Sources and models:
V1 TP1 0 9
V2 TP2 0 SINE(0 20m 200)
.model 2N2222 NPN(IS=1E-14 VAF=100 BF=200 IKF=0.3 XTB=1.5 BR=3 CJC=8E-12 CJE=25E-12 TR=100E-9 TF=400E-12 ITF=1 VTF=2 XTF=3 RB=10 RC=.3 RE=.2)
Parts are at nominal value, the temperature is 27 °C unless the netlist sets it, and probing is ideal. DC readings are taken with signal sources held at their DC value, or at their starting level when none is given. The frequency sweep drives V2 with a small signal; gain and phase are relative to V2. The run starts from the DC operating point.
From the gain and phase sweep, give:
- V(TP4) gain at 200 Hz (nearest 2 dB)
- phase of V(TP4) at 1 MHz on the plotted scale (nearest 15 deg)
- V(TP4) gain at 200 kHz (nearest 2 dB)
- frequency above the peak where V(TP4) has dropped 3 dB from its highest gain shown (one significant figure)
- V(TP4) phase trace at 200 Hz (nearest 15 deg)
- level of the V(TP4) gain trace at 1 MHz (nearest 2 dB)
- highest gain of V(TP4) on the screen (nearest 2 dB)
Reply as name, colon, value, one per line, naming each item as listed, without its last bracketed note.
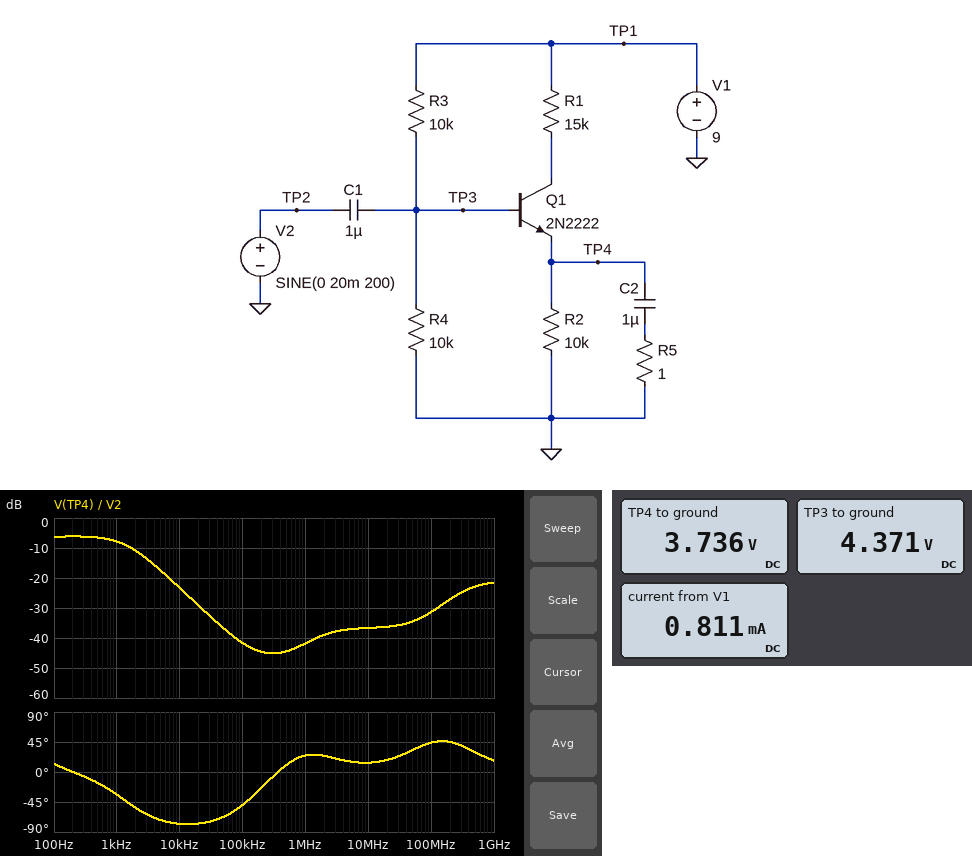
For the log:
V(TP4) gain at 200 Hz: -6 dB
phase of V(TP4) at 1 MHz on the plotted scale: 30 deg
V(TP4) gain at 200 kHz: -44 dB
frequency above the peak where V(TP4) has dropped 3 dB from its highest gain shown: 1 kHz
V(TP4) phase trace at 200 Hz: 0 deg
level of the V(TP4) gain trace at 1 MHz: -42 dB
highest gain of V(TP4) on the screen: -6 dB
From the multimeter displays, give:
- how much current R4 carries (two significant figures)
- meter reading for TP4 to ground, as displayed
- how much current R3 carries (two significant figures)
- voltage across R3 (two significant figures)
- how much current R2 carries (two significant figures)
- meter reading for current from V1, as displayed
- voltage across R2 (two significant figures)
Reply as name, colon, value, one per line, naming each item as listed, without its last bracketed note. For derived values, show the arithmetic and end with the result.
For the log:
how much current R4 carries: (4.371 V) / 10 kΩ = 440 µA
meter reading for TP4 to ground, as displayed: 3.736 V
how much current R3 carries: (9 V - 4.371 V) / 10 kΩ = 460 µA
voltage across R3: 9 V - 4.371 V = 4.6 V
how much current R2 carries: (3.736 V) / 10 kΩ = 370 µA
meter reading for current from V1, as displayed: 0.811 mA
voltage across R2: 3.736 V = 3.7 V
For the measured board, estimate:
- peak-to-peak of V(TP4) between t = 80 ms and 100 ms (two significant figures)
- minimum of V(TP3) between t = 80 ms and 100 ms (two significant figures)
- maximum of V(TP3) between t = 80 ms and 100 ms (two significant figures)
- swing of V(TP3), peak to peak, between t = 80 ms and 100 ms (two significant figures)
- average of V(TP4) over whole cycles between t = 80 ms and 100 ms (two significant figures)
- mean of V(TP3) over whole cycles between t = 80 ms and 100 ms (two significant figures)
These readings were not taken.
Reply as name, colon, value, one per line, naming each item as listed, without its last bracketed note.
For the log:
peak-to-peak of V(TP4) between t = 80 ms and 100 ms: 20 mV
minimum of V(TP3) between t = 80 ms and 100 ms: 4.4 V
maximum of V(TP3) between t = 80 ms and 100 ms: 4.4 V
swing of V(TP3), peak to peak, between t = 80 ms and 100 ms: 21 mV
average of V(TP4) over whole cycles between t = 80 ms and 100 ms: 3.7 V
mean of V(TP3) over whole cycles between t = 80 ms and 100 ms: 4.4 V
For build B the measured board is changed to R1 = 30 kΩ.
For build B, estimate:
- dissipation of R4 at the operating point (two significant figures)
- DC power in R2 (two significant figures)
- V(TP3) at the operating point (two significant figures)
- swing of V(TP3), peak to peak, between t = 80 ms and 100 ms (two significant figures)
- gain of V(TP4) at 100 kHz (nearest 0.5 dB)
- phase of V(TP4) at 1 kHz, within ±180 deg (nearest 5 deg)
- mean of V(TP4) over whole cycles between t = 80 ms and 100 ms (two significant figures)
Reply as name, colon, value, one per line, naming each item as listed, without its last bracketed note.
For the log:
dissipation of R4 at the operating point: 1.5 mW
DC power in R2: 1.0 mW
V(TP3) at the operating point: 3.9 V
swing of V(TP3), peak to peak, between t = 80 ms and 100 ms: 20 mV
gain of V(TP4) at 100 kHz: -38.5 dB
phase of V(TP4) at 1 kHz, within ±180 deg: -25 deg
mean of V(TP4) over whole cycles between t = 80 ms and 100 ms: 3.2 V
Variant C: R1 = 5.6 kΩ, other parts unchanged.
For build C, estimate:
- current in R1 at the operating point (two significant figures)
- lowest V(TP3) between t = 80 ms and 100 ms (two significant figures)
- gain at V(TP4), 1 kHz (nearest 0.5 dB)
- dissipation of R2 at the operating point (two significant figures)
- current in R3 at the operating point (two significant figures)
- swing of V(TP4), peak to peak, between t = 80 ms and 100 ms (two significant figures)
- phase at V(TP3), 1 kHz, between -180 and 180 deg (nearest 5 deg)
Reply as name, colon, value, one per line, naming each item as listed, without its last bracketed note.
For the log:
current in R1 at the operating point: 380 µA
lowest V(TP3) between t = 80 ms and 100 ms: 4.5 V
gain at V(TP4), 1 kHz: -1.0 dB
dissipation of R2 at the operating point: 1.5 mW
current in R3 at the operating point: 450 µA
swing of V(TP4), peak to peak, between t = 80 ms and 100 ms: 39 mV
phase at V(TP3), 1 kHz, between -180 and 180 deg: 0 deg
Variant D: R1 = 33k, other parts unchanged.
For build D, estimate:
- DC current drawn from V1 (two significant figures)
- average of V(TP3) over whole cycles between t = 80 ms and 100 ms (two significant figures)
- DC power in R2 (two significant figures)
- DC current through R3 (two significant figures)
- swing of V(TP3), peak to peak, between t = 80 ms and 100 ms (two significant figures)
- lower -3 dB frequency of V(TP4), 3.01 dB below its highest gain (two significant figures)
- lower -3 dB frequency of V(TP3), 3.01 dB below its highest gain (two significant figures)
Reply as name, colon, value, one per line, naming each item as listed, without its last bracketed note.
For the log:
DC current drawn from V1: 700 µA
average of V(TP3) over whole cycles between t = 80 ms and 100 ms: 3.8 V
DC power in R2: 1.0 mW
DC current through R3: 520 µA
swing of V(TP3), peak to peak, between t = 80 ms and 100 ms: 20 mV
lower -3 dB frequency of V(TP4), 3.01 dB below its highest gain: 26 Hz
lower -3 dB frequency of V(TP3), 3.01 dB below its highest gain: 1.5 kHz
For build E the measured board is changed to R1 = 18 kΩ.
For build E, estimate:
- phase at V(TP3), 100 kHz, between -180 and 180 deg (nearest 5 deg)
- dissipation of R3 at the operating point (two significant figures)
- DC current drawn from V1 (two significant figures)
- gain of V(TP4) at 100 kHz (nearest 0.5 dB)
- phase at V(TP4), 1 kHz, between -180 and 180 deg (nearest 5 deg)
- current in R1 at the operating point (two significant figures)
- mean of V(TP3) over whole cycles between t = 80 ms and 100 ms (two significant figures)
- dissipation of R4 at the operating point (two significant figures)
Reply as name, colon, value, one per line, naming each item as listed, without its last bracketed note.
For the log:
phase at V(TP3), 100 kHz, between -180 and 180 deg: 0 deg
dissipation of R3 at the operating point: 2.3 mW
DC current drawn from V1: 780 µA
gain of V(TP4) at 100 kHz: -40.5 dB
phase at V(TP4), 1 kHz, between -180 and 180 deg: -30 deg
current in R1 at the operating point: 300 µA
mean of V(TP3) over whole cycles between t = 80 ms and 100 ms: 4.2 V
dissipation of R4 at the operating point: 1.8 mW
